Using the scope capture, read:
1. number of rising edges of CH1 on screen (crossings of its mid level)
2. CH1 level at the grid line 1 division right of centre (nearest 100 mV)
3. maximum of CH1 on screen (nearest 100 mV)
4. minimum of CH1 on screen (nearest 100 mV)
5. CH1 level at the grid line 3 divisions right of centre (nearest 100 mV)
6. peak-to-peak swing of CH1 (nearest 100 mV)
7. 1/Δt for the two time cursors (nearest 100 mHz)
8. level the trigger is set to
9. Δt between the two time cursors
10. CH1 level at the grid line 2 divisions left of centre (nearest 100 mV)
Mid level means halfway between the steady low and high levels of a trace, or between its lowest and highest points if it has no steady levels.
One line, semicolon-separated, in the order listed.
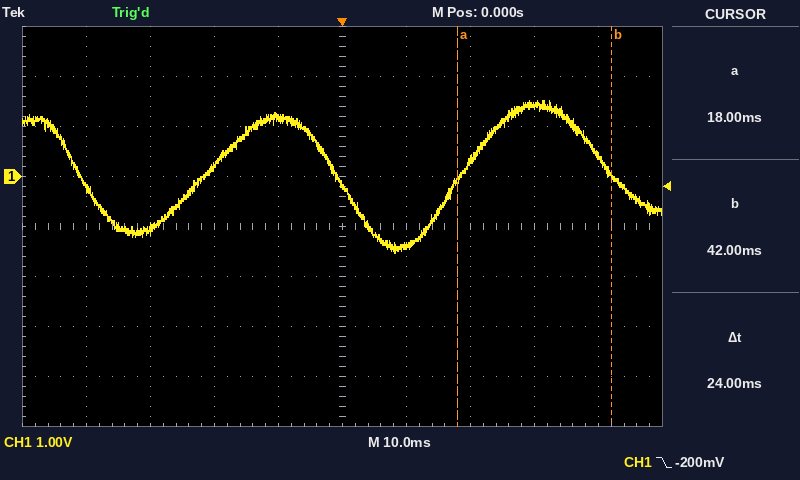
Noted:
2; -1.4 V; 1.5 V; -1.5 V; 1.4 V; 3.0 V; 41.7 Hz; -200 mV; 24 ms; 200 mV
